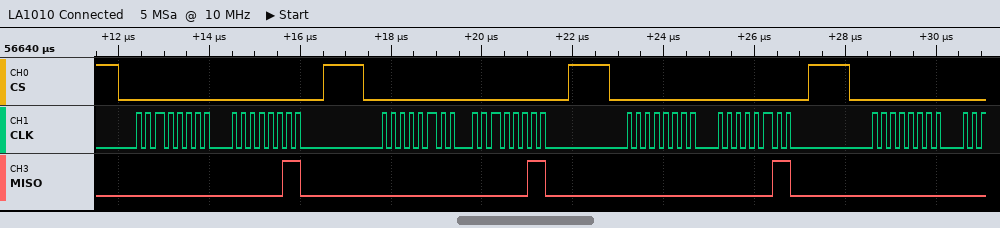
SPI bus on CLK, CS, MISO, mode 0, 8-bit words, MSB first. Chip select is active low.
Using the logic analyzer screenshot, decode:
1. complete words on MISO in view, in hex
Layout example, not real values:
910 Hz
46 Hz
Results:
00, 03, 00, 03, 00, 03, 00
